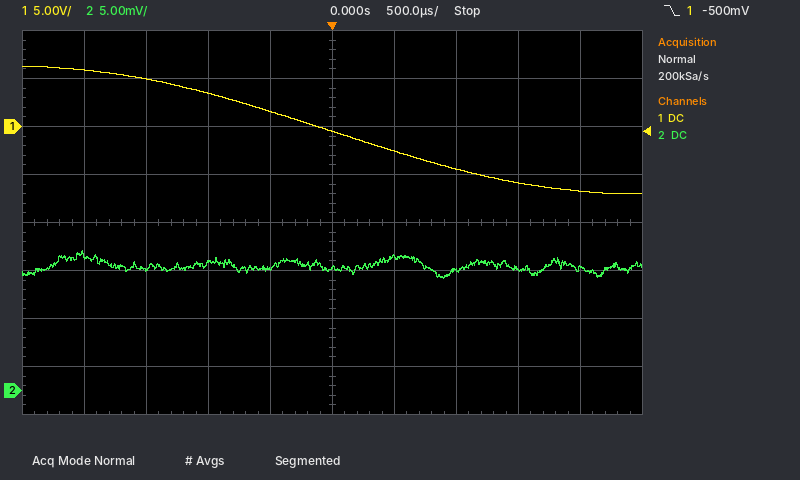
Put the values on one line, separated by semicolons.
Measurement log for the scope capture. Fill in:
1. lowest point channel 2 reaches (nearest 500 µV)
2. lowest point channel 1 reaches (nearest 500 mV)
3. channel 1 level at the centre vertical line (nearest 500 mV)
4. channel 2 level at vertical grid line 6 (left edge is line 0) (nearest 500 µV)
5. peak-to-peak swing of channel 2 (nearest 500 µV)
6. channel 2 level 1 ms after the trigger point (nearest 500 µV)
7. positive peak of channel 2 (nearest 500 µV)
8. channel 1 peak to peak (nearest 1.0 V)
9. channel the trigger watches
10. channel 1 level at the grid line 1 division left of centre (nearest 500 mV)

11.5 mV; -7.0 V; -500 mV; 14.0 mV; 3.0 mV; 12.5 mV; 14.5 mV; 13.0 V; channel 1; 1.5 V
